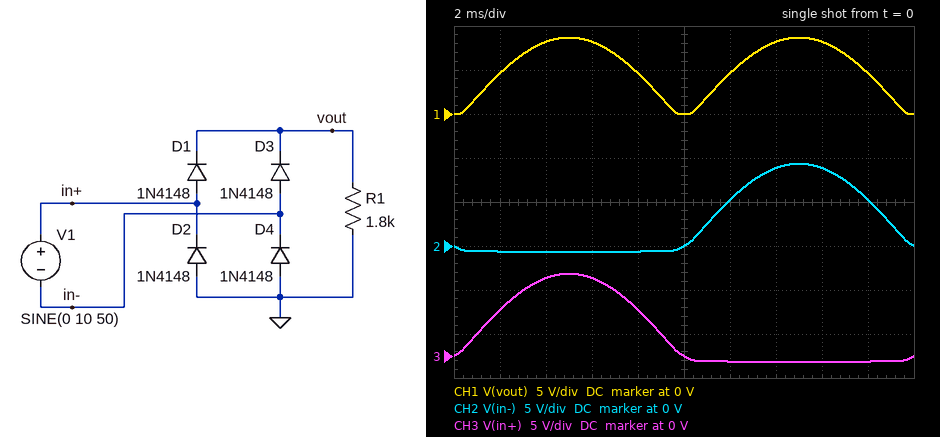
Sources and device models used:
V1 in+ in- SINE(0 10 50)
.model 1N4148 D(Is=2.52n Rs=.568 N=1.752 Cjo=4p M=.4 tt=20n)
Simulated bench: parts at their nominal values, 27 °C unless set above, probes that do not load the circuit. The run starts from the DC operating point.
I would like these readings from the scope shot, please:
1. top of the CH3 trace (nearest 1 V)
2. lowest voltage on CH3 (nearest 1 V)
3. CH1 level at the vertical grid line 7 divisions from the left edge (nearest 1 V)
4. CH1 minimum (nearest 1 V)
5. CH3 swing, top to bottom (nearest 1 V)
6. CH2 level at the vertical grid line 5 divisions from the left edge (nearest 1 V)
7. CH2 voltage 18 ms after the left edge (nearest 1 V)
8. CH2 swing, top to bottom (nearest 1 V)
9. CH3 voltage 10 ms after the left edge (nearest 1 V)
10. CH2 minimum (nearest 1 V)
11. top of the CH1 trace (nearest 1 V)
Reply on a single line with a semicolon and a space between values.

9 V; -1 V; 8 V; 0 V; 10 V; 0 V; 5 V; 10 V; 0 V; -1 V; 9 V
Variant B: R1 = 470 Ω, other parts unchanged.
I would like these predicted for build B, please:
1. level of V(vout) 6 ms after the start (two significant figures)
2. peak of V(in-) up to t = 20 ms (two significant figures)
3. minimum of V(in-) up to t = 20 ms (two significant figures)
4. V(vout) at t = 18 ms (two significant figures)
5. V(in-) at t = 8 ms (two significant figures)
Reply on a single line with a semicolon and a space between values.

8.1 V; 9.3 V; -730 mV; 4.5 V; -690 mV
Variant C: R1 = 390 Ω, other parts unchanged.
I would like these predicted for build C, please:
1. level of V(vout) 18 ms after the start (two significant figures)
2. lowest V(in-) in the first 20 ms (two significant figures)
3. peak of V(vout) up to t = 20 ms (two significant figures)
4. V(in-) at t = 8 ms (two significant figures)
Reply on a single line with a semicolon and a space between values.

4.5 V; -740 mV; 8.5 V; -700 mV
